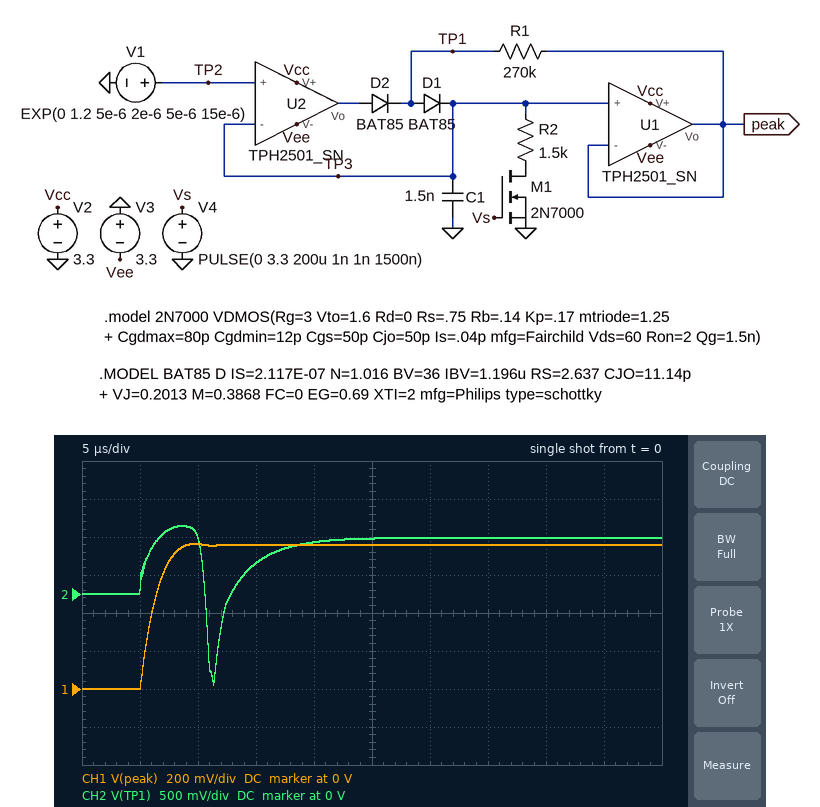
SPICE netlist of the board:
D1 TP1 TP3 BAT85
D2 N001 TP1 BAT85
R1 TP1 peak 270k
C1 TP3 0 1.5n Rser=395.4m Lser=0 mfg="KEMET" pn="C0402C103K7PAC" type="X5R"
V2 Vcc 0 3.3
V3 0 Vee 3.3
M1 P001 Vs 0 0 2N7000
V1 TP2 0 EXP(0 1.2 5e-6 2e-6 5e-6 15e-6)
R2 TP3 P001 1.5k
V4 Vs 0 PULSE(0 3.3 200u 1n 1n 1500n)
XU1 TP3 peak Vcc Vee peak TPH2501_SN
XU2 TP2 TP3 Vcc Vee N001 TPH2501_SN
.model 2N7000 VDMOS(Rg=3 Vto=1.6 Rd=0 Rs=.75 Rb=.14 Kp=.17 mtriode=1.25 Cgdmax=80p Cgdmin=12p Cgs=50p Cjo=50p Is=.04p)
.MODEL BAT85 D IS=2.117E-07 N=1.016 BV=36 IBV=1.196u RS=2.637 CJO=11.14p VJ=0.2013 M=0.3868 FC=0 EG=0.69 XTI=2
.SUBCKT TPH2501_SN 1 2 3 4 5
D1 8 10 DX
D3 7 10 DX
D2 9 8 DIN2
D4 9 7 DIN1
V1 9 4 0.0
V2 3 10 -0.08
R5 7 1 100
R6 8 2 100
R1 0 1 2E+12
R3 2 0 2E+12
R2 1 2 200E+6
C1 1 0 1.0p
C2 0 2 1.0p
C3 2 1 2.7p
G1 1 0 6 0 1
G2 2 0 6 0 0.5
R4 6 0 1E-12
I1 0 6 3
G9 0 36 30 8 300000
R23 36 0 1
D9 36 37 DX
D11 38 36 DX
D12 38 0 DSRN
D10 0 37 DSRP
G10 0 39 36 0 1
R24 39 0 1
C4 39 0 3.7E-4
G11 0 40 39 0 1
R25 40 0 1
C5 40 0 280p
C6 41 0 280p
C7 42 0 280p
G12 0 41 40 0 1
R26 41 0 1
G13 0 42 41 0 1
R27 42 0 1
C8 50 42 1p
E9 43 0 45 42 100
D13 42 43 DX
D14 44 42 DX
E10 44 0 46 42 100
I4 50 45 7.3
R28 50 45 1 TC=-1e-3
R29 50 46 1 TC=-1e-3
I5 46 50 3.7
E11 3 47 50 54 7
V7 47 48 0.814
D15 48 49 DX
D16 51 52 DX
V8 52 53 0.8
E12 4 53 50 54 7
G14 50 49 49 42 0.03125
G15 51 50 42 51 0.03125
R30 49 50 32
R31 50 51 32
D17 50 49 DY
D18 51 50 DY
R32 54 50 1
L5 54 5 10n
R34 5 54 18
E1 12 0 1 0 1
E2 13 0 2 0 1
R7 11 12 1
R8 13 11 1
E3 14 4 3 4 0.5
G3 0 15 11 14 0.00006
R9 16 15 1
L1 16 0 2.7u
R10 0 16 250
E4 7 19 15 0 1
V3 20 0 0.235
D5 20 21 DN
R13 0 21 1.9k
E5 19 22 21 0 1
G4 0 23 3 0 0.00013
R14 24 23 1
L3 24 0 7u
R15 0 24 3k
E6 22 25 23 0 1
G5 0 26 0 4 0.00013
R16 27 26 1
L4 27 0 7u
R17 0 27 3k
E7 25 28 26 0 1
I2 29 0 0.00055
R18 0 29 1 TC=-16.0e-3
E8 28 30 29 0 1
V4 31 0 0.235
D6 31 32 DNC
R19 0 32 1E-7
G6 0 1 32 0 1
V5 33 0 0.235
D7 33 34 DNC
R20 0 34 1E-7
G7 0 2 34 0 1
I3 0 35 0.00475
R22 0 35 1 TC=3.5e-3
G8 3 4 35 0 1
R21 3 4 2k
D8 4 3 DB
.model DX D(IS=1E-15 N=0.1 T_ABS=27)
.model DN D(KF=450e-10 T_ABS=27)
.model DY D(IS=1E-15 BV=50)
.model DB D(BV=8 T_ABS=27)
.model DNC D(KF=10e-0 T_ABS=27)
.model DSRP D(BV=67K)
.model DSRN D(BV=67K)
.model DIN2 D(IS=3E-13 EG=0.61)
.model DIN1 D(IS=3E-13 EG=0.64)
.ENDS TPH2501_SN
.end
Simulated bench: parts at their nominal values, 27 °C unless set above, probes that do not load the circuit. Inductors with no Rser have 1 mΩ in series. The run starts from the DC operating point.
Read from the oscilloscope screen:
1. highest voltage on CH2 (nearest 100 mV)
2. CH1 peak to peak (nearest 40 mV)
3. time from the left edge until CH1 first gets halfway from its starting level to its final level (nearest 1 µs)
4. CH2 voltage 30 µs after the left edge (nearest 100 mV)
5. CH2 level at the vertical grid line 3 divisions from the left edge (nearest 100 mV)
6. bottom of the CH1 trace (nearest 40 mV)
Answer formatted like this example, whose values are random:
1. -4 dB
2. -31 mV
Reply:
1. 900 mV
2. 760 mV
3. 6 µs
4. 700 mV
5. 400 mV
6. 0 V
